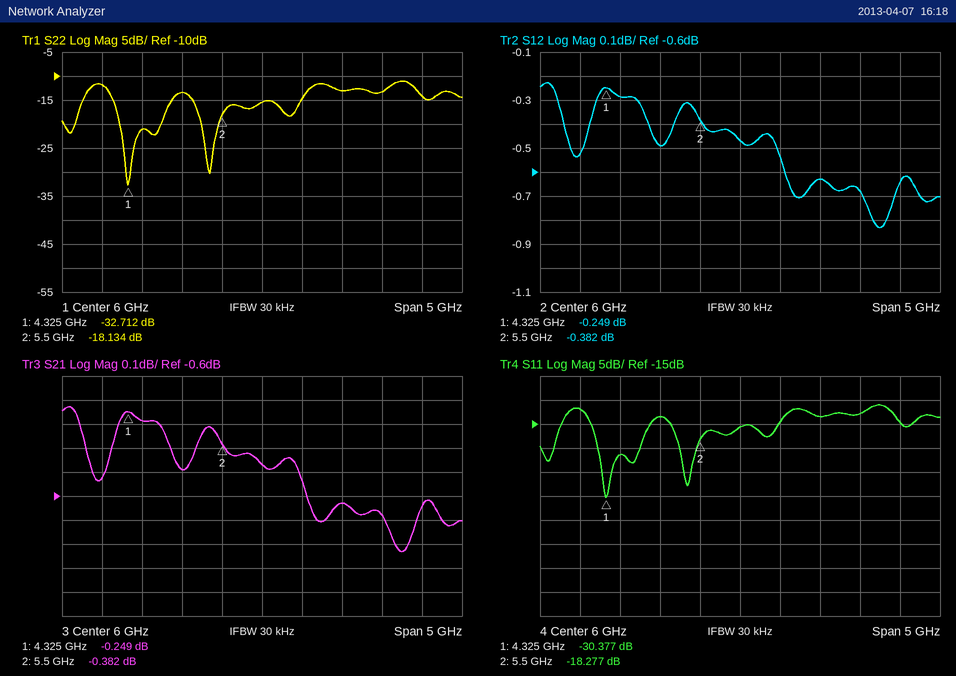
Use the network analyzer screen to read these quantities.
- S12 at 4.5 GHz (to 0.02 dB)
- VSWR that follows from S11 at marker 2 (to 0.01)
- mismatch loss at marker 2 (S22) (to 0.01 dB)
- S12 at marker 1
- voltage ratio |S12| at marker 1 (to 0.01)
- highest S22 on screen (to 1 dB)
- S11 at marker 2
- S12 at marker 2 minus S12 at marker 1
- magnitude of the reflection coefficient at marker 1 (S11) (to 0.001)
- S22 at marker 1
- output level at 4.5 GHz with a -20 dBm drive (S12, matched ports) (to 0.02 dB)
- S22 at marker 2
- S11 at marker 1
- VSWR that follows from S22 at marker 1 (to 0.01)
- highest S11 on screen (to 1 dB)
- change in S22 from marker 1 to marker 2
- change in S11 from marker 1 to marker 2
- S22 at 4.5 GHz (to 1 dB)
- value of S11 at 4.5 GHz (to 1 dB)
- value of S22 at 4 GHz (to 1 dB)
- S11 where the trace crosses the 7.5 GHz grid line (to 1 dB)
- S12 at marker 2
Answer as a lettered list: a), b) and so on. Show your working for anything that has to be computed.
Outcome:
a) -0.28 dB
b) (1 + 0.1219)/(1 − 0.1219) ≈ 1.28
c) −10 log10(1 − 10^(-18.134/10)) ≈ 0.07 dB
d) -0.249 dB
e) 10^(-0.249/20) ≈ 0.97
f) -11 dB
g) -18.277 dB
h) -0.382 − (-0.249) = -0.133 dB
i) 10^(-30.377/20) ≈ 0.030
j) -32.712 dB
k) -20 dBm + (-0.28 dB) = -20.28 dBm
l) -18.134 dB
m) -30.377 dB
n) (1 + 0.0231)/(1 − 0.0231) ≈ 1.05
o) -11 dB
p) -18.134 − (-32.712) = 14.578 dB
q) -18.277 − (-30.377) = 12.100 dB
r) -21 dB
s) -21 dB
t) -12 dB
u) -13 dB
v) -0.382 dB
